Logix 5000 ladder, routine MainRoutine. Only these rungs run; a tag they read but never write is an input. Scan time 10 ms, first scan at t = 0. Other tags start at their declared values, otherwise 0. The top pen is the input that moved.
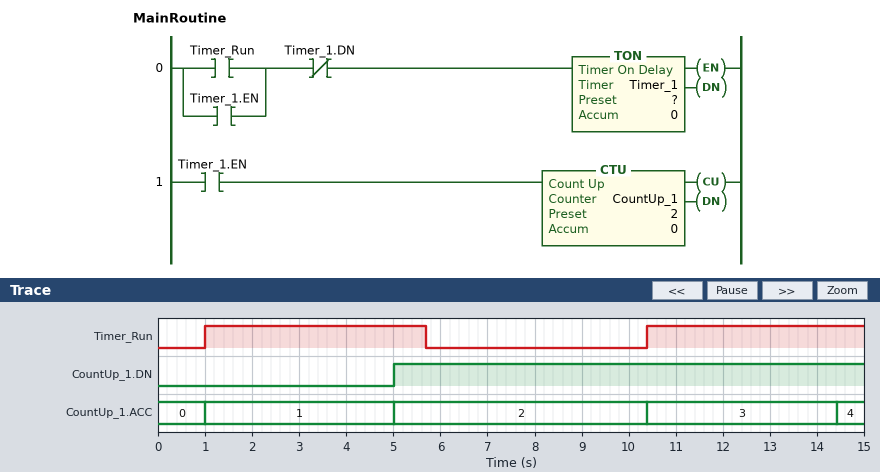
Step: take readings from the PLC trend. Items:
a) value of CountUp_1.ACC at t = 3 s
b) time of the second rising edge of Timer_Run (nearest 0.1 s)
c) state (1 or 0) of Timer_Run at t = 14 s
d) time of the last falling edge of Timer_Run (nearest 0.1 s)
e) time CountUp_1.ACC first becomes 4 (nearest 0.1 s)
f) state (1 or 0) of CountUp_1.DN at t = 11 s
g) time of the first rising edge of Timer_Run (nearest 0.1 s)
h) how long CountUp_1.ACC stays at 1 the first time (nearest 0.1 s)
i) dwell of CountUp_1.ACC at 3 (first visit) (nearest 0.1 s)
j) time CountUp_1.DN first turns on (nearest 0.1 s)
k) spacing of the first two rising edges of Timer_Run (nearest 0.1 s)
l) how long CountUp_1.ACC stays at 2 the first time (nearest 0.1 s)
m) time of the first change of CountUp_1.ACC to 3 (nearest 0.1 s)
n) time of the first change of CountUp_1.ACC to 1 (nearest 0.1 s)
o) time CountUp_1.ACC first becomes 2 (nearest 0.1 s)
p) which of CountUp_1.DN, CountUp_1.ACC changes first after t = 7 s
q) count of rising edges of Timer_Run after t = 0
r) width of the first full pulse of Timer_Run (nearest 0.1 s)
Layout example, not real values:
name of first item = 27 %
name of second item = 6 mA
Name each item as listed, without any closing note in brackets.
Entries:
value of CountUp_1.ACC at t = 3 s = 1
time of the second rising edge of Timer_Run = 10.4 s
state (1 or 0) of Timer_Run at t = 14 s = 1
time of the last falling edge of Timer_Run = 5.7 s
time CountUp_1.ACC first becomes 4 = 14.4 s
state (1 or 0) of CountUp_1.DN at t = 11 s = 1
time of the first rising edge of Timer_Run = 1.0 s
how long CountUp_1.ACC stays at 1 the first time = 4.0 s
dwell of CountUp_1.ACC at 3 (first visit) = 4.0 s
time CountUp_1.DN first turns on = 5.0 s
spacing of the first two rising edges of Timer_Run = 9.4 s
how long CountUp_1.ACC stays at 2 the first time = 5.4 s
time of the first change of CountUp_1.ACC to 3 = 10.4 s
time of the first change of CountUp_1.ACC to 1 = 1.0 s
time CountUp_1.ACC first becomes 2 = 5.0 s
which of CountUp_1.DN, CountUp_1.ACC changes first after t = 7 s = CountUp_1.ACC
count of rising edges of Timer_Run after t = 0 = 2
width of the first full pulse of Timer_Run = 4.7 s
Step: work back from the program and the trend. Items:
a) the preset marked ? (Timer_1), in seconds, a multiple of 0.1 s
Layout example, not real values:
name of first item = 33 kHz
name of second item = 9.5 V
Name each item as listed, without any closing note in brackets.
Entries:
the preset marked ? (Timer_1), in seconds, a multiple of 0.1 s = 4.0 s
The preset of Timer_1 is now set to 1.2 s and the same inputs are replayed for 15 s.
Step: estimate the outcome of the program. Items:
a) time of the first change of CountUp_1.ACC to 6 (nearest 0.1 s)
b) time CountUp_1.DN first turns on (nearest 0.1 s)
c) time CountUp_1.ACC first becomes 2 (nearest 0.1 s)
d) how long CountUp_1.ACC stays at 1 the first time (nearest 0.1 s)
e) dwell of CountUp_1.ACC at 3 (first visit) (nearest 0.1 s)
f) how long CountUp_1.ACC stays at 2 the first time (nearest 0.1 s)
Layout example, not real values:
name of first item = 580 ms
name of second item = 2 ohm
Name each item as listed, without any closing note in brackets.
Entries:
time of the first change of CountUp_1.ACC to 6 = 11.6 s
time CountUp_1.DN first turns on = 2.2 s
time CountUp_1.ACC first becomes 2 = 2.2 s
how long CountUp_1.ACC stays at 1 the first time = 1.2 s
dwell of CountUp_1.ACC at 3 (first visit) = 1.2 s
how long CountUp_1.ACC stays at 2 the first time = 1.2 s
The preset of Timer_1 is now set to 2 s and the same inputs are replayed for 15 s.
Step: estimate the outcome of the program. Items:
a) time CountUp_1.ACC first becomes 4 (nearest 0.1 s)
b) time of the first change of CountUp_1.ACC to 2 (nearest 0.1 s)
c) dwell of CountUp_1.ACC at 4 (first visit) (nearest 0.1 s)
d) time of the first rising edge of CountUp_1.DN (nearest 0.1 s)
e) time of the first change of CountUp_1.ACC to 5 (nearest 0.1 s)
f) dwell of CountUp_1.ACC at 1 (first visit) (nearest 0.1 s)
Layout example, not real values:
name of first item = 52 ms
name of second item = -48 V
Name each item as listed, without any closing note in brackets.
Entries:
time CountUp_1.ACC first becomes 4 = 10.4 s
time of the first change of CountUp_1.ACC to 2 = 3.0 s
dwell of CountUp_1.ACC at 4 (first visit) = 2.0 s
time of the first rising edge of CountUp_1.DN = 3.0 s
time of the first change of CountUp_1.ACC to 5 = 12.4 s
dwell of CountUp_1.ACC at 1 (first visit) = 2.0 s
